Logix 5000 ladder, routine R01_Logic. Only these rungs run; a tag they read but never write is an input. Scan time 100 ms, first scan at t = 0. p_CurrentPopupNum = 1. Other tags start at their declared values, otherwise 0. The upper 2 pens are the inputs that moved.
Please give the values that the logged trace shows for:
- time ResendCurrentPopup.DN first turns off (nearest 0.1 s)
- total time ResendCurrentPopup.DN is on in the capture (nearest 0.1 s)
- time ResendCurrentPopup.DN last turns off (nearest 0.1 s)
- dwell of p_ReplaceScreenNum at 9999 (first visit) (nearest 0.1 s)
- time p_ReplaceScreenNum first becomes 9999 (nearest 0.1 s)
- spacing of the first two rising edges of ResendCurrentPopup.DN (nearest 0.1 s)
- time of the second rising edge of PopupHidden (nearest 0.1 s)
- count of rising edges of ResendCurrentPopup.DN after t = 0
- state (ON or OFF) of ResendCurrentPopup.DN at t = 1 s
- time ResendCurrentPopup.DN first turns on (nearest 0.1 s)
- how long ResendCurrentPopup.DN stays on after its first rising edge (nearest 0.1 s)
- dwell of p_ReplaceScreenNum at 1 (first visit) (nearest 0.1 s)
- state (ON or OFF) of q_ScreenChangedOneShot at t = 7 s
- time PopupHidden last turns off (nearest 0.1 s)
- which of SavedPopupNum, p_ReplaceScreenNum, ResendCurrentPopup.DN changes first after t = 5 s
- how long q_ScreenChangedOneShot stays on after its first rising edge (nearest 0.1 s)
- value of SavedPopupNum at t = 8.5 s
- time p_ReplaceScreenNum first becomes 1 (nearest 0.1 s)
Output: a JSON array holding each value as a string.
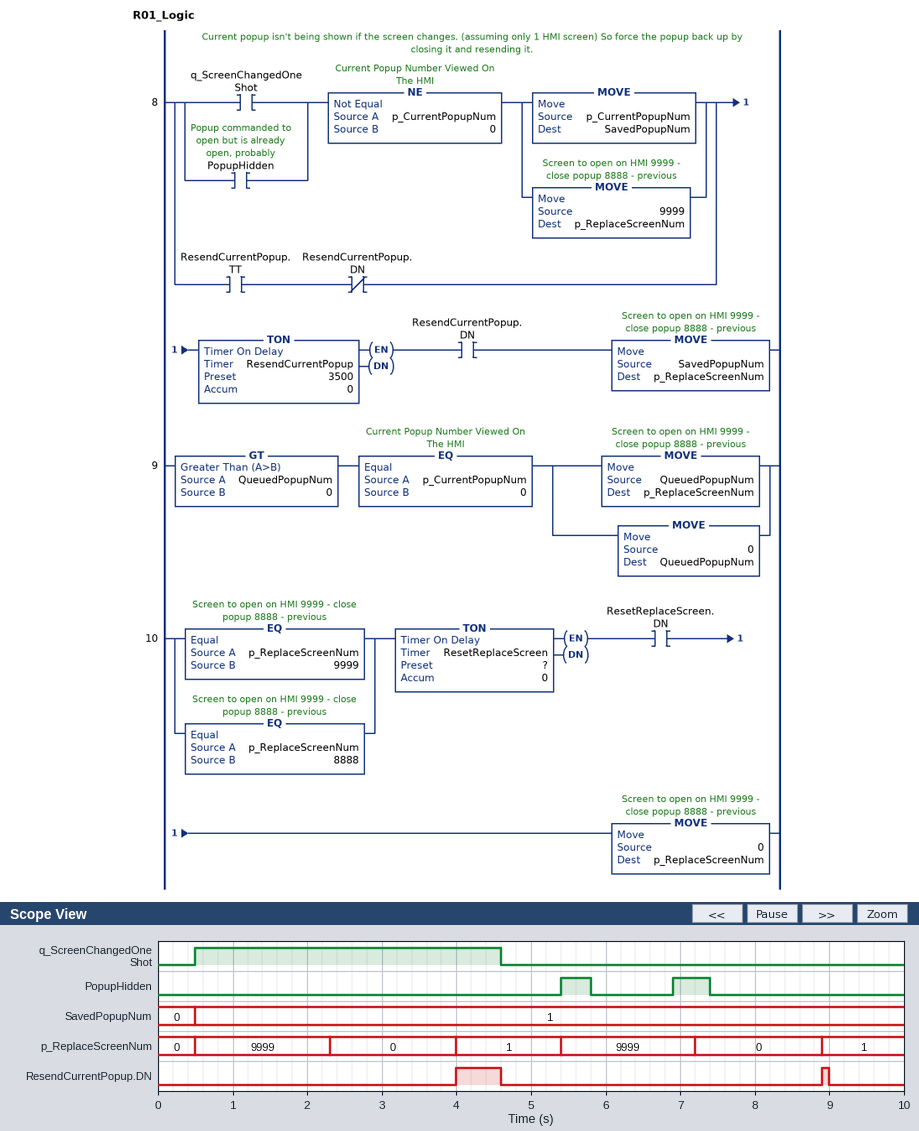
["4.6 s", "0.7 s", "9.0 s", "1.8 s", "0.5 s", "4.9 s", "6.9 s", "2", "OFF", "4.0 s", "0.6 s", "1.4 s", "OFF", "7.4 s", "p_ReplaceScreenNum", "4.1 s", "1", "4.0 s"]
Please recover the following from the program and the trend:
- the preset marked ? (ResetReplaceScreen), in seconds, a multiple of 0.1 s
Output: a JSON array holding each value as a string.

["1.8 s"]
